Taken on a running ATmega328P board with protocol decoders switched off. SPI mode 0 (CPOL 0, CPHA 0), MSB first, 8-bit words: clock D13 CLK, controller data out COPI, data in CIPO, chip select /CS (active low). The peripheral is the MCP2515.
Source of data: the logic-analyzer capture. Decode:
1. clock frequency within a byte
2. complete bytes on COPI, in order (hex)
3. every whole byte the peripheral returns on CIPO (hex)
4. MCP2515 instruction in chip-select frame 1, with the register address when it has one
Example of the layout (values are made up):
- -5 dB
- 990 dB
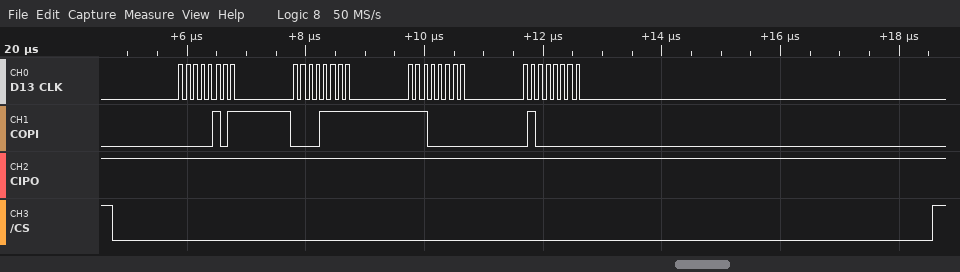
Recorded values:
- 8 MHz
- 0x05 0x0F 0xE0 0x40
- 0xFF 0xFF 0xFF 0xFF
- BIT MODIFY 0x0F
